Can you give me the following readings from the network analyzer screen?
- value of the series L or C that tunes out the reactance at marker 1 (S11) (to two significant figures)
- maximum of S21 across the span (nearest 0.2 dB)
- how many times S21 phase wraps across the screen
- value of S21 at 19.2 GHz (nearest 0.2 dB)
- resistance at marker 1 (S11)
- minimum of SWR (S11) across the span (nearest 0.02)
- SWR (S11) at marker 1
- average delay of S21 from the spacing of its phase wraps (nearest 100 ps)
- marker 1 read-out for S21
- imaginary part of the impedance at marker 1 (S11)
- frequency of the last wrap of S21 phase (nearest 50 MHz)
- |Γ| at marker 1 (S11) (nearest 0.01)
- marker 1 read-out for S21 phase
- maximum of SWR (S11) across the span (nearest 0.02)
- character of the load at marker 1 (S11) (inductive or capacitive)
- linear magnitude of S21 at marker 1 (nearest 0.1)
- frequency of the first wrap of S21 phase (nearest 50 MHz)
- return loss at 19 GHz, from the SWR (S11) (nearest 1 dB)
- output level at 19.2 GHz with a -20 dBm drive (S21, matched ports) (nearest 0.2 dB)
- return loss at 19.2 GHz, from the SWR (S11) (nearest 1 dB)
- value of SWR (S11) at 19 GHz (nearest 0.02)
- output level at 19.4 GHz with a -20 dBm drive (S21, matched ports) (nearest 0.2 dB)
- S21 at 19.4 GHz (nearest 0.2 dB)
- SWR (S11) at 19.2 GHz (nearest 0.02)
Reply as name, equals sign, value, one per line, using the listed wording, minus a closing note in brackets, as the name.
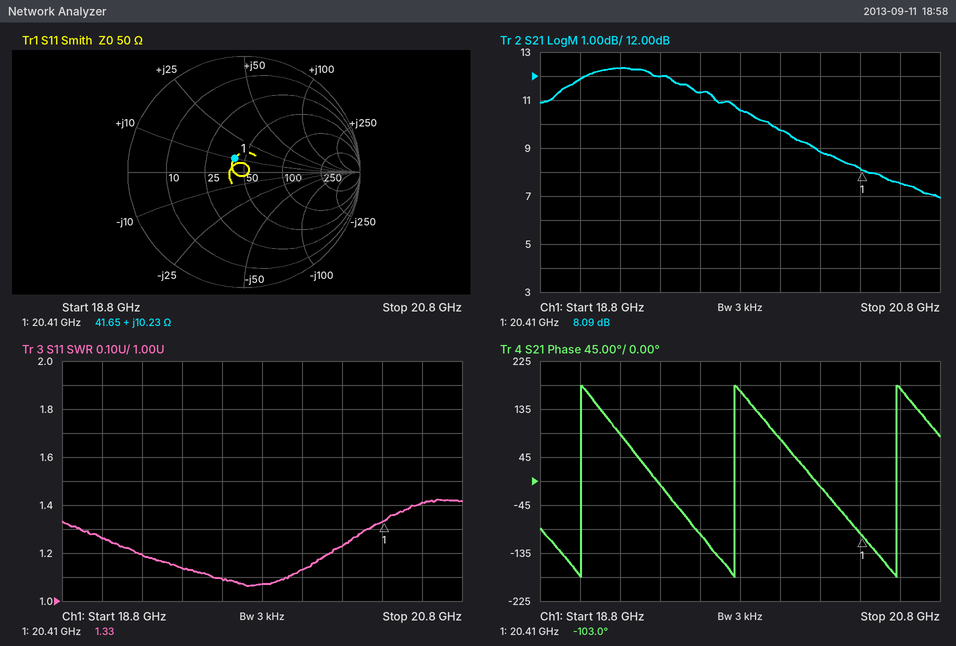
value of the series L or C that tunes out the reactance at marker 1 (S11) = 760 fF
maximum of S21 across the span = 12.4 dB
how many times S21 phase wraps across the screen = 3
value of S21 at 19.2 GHz = 12.4 dB
resistance at marker 1 = 41.65 Ω
minimum of SWR (S11) across the span = 1.06
SWR (S11) at marker 1 = 1.33
average delay of S21 from the spacing of its phase wraps = 1.3 ns
marker 1 read-out for S21 = 8.09 dB
imaginary part of the impedance at marker 1 = +10.23 Ω
frequency of the last wrap of S21 phase = 20.60 GHz
|Γ| at marker 1 (S11) = 0.14
marker 1 read-out for S21 phase = -103.0°
maximum of SWR (S11) across the span = 1.42
character of the load at marker 1 (S11) = inductive
linear magnitude of S21 at marker 1 = 2.5
frequency of the first wrap of S21 phase = 19.00 GHz
return loss at 19 GHz, from the SWR (S11) = 19 dB
output level at 19.2 GHz with a -20 dBm drive (S21, matched ports) = -7.6 dBm
return loss at 19.2 GHz, from the SWR (S11) = 21 dB
value of SWR (S11) at 19 GHz = 1.26
output level at 19.4 GHz with a -20 dBm drive (S21, matched ports) = -8.0 dBm
S21 at 19.4 GHz = 12.0 dB
SWR (S11) at 19.2 GHz = 1.20
